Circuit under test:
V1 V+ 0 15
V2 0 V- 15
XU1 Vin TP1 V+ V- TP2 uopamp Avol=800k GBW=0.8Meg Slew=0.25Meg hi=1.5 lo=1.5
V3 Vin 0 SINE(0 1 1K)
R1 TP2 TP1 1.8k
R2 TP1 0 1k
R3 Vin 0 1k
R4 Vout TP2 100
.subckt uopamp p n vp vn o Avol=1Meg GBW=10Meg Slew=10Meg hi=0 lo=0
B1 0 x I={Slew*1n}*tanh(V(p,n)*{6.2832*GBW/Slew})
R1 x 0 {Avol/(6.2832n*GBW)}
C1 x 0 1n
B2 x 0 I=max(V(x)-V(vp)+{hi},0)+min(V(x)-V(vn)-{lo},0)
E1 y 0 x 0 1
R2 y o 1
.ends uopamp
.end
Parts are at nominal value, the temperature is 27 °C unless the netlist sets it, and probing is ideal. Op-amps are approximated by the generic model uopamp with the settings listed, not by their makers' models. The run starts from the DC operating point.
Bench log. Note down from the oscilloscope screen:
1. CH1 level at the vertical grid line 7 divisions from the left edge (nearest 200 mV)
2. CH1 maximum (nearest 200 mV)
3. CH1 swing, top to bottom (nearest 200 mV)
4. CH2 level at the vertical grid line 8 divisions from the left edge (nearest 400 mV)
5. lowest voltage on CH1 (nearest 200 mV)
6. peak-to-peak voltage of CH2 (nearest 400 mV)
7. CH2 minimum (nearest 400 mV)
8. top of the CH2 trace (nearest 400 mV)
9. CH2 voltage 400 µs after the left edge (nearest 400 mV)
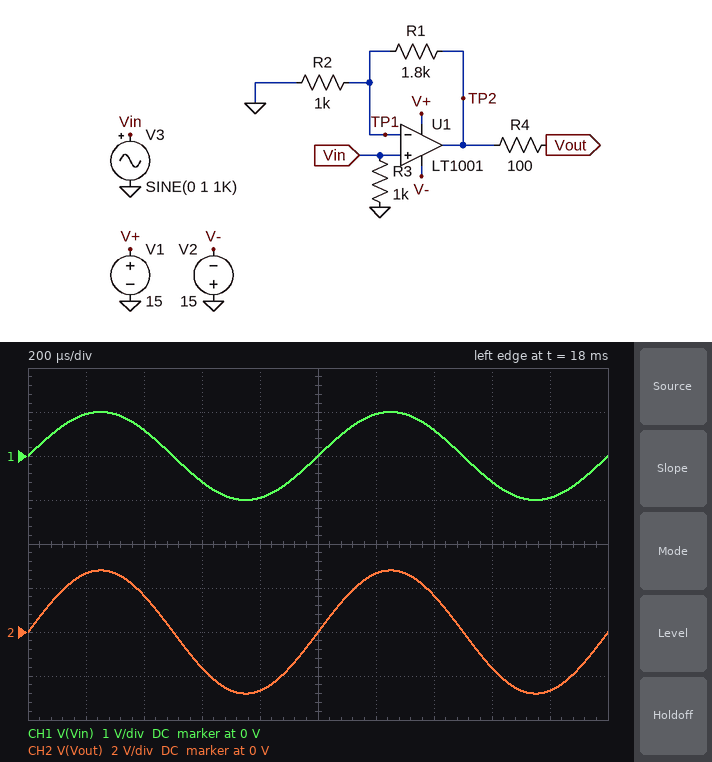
600 mV
1.0 V
2.0 V
-1.6 V
-1.0 V
5.6 V
-2.8 V
2.8 V
1.6 V
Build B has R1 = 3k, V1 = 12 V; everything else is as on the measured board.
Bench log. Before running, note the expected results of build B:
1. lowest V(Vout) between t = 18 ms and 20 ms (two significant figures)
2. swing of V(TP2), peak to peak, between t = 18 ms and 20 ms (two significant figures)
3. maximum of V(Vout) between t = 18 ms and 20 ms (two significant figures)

-4.0 V
8.0 V
4.0 V
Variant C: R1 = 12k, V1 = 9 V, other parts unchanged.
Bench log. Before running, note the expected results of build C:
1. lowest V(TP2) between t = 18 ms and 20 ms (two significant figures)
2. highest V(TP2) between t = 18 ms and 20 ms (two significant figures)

-13 V
7.5 V
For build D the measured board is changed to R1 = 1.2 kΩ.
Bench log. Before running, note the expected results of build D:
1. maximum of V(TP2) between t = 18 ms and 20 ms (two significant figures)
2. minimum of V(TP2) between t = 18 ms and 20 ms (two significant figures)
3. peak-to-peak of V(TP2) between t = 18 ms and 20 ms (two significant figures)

2.2 V
-2.2 V
4.4 V
